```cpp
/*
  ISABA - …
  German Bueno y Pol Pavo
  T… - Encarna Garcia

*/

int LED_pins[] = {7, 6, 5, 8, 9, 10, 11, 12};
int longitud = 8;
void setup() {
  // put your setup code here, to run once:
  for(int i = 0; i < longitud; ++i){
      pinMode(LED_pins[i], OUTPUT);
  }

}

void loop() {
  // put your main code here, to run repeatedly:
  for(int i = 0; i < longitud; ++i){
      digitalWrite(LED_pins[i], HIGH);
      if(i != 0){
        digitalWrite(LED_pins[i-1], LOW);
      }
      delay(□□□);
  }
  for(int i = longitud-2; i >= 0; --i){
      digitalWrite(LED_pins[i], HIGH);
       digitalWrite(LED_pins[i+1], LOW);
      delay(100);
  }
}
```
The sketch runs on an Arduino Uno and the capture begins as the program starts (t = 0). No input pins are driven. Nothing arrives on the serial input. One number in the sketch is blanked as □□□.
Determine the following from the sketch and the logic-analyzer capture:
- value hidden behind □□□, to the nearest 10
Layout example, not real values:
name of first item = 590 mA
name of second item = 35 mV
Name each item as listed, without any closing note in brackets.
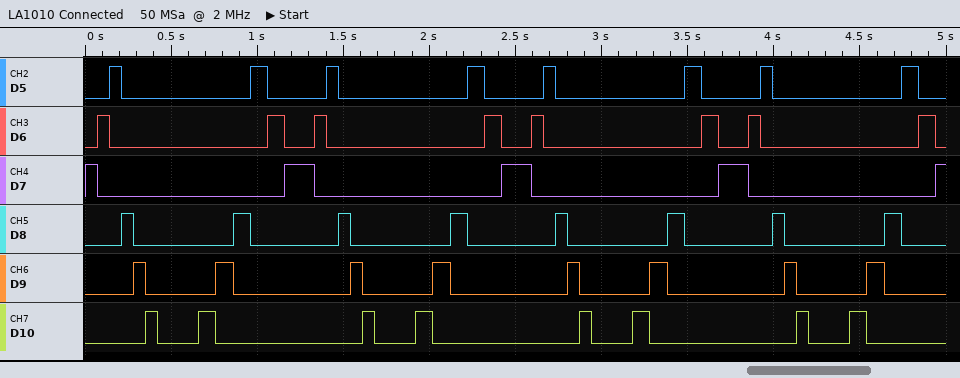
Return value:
value hidden behind □□□, to the nearest 10 = 70
